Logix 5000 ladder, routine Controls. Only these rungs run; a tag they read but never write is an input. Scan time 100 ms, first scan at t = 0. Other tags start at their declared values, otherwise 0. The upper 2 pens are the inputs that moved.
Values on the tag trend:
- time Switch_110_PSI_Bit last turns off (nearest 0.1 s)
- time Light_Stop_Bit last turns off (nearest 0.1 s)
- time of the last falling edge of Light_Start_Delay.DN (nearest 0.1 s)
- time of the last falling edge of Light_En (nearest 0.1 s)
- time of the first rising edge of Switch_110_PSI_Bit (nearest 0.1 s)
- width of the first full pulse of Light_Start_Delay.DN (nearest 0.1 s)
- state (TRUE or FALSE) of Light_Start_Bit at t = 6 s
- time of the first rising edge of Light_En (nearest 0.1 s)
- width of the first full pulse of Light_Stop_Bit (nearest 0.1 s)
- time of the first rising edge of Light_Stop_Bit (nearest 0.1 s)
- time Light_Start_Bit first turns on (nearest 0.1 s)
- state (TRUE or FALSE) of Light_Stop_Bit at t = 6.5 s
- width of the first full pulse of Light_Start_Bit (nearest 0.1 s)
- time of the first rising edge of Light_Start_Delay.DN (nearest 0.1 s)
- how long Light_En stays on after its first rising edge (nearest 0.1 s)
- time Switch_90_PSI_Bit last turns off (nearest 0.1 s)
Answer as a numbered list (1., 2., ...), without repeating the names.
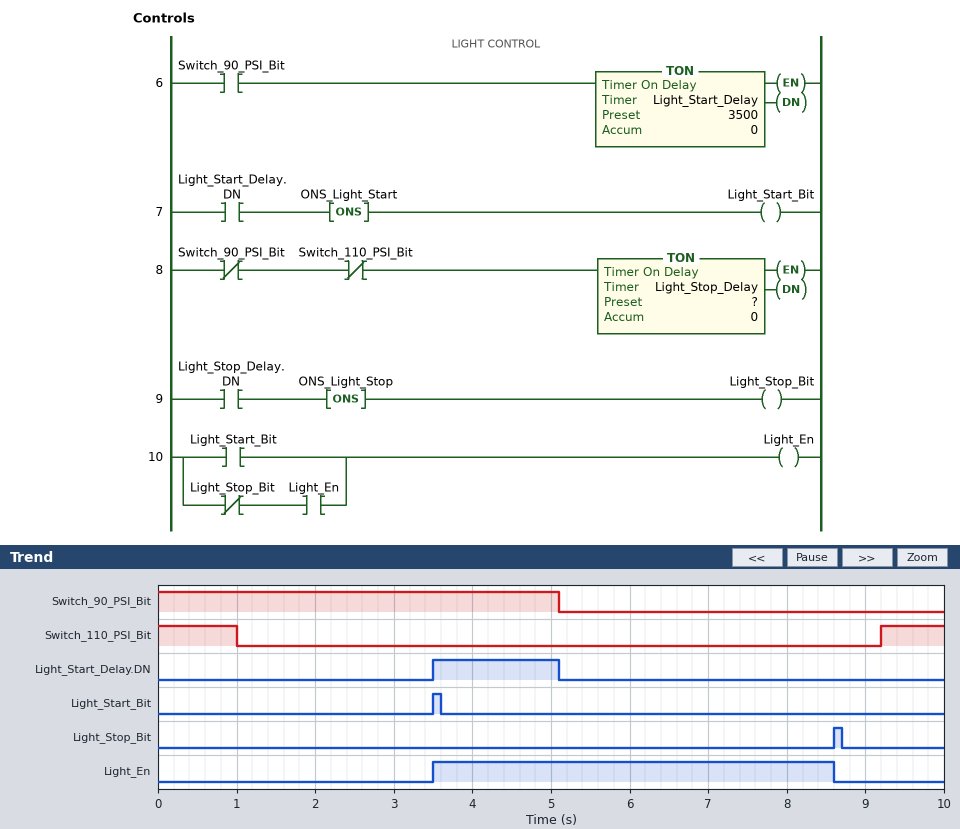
1. 1.0 s
2. 8.7 s
3. 5.1 s
4. 8.6 s
5. 9.2 s
6. 1.6 s
7. FALSE
8. 3.5 s
9. 0.1 s
10. 8.6 s
11. 3.5 s
12. FALSE
13. 0.1 s
14. 3.5 s
15. 5.1 s
16. 5.1 s
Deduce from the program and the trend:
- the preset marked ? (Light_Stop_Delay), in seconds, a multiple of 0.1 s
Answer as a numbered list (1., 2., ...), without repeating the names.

1. 3.5 s
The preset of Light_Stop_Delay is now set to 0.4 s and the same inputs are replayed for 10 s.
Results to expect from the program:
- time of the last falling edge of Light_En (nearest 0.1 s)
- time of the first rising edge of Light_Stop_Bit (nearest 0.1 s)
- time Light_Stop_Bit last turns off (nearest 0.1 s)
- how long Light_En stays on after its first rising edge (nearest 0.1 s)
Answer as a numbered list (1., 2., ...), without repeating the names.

1. 5.5 s
2. 5.5 s
3. 5.6 s
4. 2.0 s
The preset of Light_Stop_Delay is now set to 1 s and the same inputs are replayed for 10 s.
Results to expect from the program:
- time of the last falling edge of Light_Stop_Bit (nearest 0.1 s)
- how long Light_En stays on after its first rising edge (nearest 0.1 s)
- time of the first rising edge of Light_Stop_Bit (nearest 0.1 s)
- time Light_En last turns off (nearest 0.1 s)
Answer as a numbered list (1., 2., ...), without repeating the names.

1. 6.2 s
2. 2.6 s
3. 6.1 s
4. 6.1 s
